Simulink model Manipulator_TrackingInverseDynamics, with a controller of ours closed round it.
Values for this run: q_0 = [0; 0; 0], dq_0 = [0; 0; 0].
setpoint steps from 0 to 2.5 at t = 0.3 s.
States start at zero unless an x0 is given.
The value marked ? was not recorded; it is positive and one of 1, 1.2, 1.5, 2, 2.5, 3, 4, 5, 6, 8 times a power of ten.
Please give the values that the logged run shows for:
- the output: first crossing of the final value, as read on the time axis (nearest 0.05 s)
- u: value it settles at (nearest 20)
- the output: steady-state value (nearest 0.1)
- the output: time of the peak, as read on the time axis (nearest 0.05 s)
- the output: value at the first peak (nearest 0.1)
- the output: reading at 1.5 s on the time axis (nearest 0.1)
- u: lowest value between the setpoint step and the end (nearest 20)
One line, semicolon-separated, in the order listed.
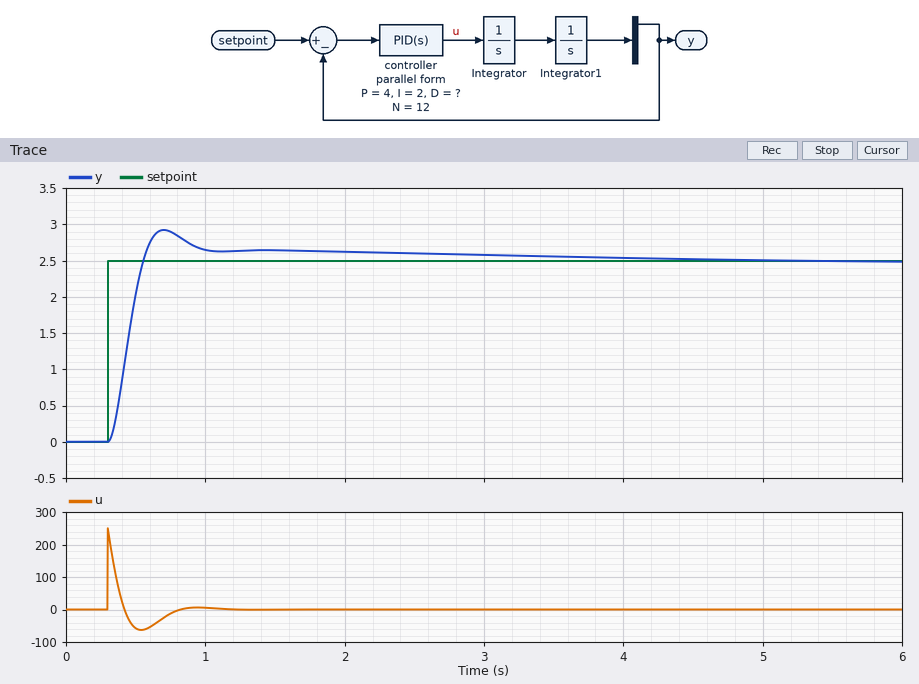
0.55 s; 0; 2.5; 0.70 s; 2.9; 2.6; -60
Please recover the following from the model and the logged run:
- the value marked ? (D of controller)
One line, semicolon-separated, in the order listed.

8
